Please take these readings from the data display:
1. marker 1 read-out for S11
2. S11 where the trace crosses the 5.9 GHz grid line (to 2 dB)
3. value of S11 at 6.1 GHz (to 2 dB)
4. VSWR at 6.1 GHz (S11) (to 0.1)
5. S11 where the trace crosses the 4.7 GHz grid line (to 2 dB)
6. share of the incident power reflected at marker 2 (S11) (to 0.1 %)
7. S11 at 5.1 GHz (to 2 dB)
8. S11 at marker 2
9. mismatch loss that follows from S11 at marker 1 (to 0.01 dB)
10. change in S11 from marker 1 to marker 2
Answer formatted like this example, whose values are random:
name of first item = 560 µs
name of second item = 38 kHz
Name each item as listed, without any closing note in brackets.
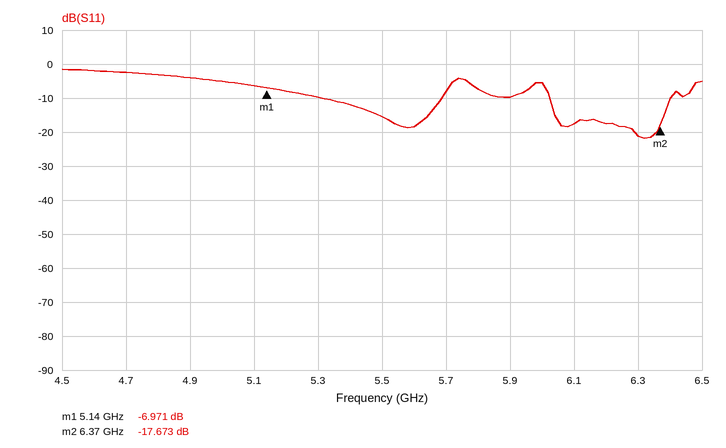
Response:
marker 1 read-out for S11 = -6.971 dB
S11 where the trace crosses the 5.9 GHz grid line = -10 dB
value of S11 at 6.1 GHz = -18 dB
VSWR at 6.1 GHz (S11) = 1.3
S11 where the trace crosses the 4.7 GHz grid line = -2 dB
share of the incident power reflected at marker 2 (S11) = 1.7 %
S11 at 5.1 GHz = -6 dB
S11 at marker 2 = -17.673 dB
mismatch loss that follows from S11 at marker 1 = 0.97 dB
change in S11 from marker 1 to marker 2 = -10.702 dB
